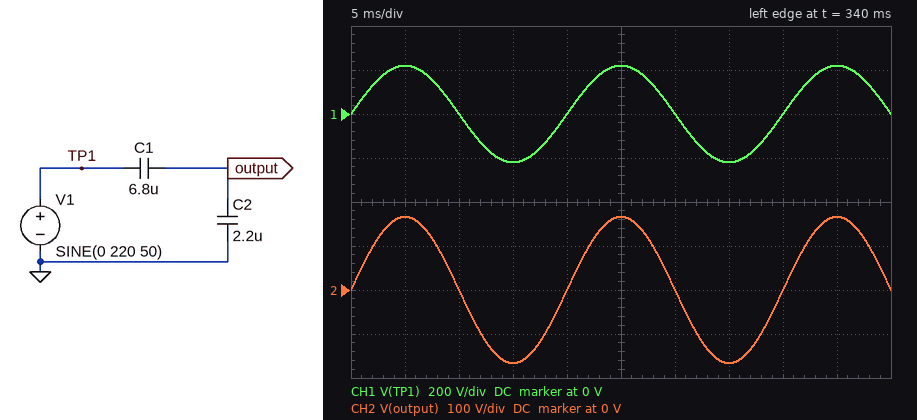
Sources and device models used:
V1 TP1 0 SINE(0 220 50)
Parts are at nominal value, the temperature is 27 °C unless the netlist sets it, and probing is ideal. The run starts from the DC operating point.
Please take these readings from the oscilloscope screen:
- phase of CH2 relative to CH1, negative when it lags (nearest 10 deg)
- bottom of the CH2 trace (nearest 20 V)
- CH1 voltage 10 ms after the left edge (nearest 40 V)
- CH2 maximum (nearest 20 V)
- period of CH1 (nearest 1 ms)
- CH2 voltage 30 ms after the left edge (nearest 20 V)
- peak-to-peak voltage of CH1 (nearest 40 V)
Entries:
0 deg
-160 V
0 V
160 V
20 ms
0 V
440 V
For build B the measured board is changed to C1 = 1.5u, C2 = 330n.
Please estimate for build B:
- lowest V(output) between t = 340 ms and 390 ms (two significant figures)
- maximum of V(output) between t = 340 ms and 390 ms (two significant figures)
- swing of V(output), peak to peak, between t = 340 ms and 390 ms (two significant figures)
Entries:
-180 V
180 V
360 V
